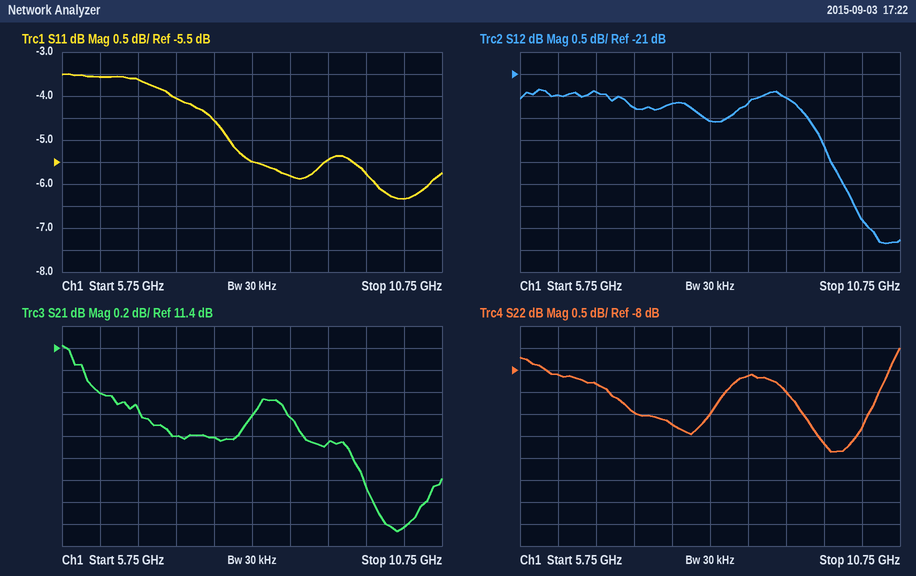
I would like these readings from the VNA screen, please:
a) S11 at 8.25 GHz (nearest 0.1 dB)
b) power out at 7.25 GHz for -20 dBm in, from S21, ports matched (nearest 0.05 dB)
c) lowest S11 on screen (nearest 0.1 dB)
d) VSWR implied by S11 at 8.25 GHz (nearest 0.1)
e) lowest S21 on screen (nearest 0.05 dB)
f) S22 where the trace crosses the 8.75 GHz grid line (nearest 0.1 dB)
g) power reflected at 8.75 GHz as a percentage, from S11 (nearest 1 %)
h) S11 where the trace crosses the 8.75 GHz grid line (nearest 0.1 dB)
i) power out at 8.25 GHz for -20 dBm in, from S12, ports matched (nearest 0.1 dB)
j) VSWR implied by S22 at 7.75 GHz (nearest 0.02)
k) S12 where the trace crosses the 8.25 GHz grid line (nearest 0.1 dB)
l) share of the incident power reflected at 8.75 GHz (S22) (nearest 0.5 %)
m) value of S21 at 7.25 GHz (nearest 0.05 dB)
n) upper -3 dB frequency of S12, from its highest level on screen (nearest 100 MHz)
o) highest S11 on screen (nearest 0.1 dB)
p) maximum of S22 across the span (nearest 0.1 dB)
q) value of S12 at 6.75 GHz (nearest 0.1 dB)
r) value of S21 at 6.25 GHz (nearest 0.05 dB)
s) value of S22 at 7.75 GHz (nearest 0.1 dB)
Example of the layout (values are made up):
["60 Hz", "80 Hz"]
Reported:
["-5.5 dB", "-9.40 dBm", "-6.3 dB", "3.3", "9.75 dB", "-8.1 dB", "26 %", "-5.8 dB", "-42.1 dBm", "2.06", "-22.1 dB", "15.5 %", "10.60 dB", "10.3 GHz", "-3.5 dB", "-7.5 dB", "-21.4 dB", "11.00 dB", "-9.2 dB"]
